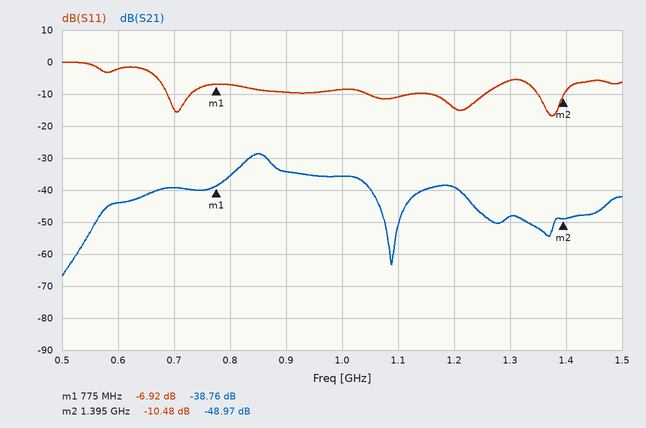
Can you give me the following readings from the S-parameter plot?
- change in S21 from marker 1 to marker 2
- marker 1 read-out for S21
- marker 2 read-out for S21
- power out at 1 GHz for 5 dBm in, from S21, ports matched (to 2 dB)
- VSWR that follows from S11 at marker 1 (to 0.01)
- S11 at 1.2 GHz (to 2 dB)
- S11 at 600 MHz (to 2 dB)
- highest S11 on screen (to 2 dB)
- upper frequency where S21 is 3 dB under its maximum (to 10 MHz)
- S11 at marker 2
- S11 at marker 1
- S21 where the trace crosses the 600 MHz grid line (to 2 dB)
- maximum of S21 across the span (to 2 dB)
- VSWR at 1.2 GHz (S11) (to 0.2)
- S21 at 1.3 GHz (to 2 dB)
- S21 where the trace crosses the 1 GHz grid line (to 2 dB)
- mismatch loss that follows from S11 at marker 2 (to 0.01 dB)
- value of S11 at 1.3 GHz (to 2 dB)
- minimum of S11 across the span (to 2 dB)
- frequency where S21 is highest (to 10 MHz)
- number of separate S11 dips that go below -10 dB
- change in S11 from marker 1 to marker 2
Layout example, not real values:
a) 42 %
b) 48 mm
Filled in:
a) -10.21 dB
b) -38.76 dB
c) -48.97 dB
d) -30 dBm
e) 2.64
f) -14 dB
g) -2 dB
h) 0 dB
i) 870 MHz
j) -10.48 dB
k) -6.92 dB
l) -44 dB
m) -28 dB
n) 1.4
o) -48 dB
p) -36 dB
q) 0.41 dB
r) -6 dB
s) -16 dB
t) 850 MHz
u) 3
v) -3.56 dB
